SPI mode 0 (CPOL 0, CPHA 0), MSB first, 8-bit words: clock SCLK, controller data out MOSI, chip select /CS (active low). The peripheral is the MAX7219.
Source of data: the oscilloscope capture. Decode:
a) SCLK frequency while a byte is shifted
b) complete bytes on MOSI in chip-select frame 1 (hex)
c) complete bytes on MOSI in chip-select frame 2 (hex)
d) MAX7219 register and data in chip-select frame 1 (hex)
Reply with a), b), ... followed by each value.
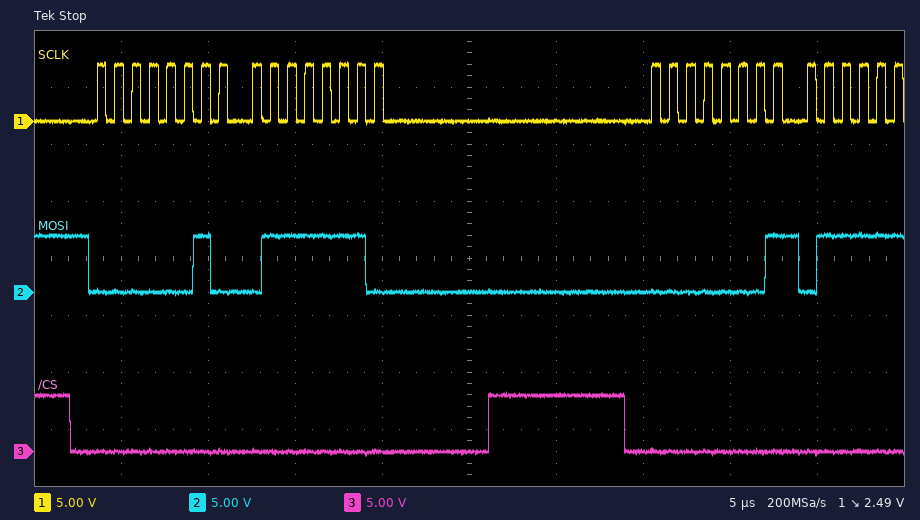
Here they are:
a) 1 MHz
b) 02 7E
c) 01
d) register 0x2, data 0x7E
